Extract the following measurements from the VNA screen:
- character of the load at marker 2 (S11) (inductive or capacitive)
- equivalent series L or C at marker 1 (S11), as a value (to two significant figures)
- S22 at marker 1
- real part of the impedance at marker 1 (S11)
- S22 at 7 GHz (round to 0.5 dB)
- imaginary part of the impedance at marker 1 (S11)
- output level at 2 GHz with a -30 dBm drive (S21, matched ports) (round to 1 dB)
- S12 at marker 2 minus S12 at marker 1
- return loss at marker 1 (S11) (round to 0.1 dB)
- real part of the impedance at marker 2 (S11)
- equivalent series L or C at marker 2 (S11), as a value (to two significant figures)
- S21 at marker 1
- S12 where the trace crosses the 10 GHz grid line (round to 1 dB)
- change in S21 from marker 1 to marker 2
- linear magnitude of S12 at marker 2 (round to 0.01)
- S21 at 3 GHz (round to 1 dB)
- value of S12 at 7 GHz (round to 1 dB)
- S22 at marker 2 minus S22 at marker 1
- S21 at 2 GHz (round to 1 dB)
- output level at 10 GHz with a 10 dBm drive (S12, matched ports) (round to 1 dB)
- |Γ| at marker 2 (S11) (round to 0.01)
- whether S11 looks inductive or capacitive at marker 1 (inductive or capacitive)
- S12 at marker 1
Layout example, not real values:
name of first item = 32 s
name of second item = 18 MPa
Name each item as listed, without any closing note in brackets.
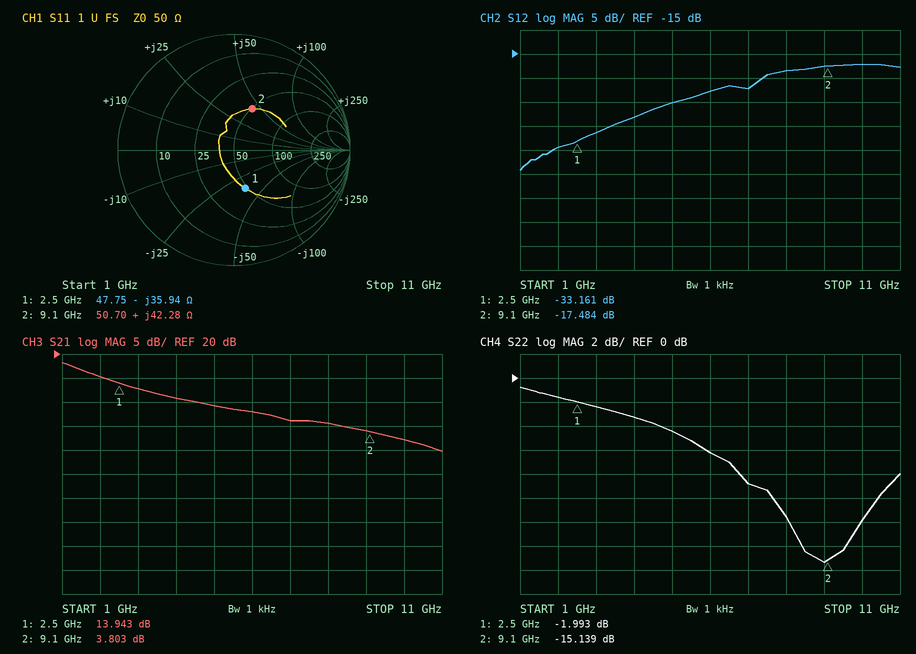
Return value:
character of the load at marker 2 (S11) = inductive
equivalent series L or C at marker 1 (S11), as a value = 1.8 pF
S22 at marker 1 = -1.993 dB
real part of the impedance at marker 1 = 47.75 Ω
S22 at 7 GHz = -9.0 dB
imaginary part of the impedance at marker 1 = -35.94 Ω
output level at 2 GHz with a -30 dBm drive (S21, matched ports) = -15 dBm
S12 at marker 2 minus S12 at marker 1 = 15.677 dB
return loss at marker 1 (S11) = 9.2 dB
real part of the impedance at marker 2 = 50.70 Ω
equivalent series L or C at marker 2 (S11), as a value = 740 pH
S21 at marker 1 = 13.943 dB
S12 where the trace crosses the 10 GHz grid line = -17 dB
change in S21 from marker 1 to marker 2 = -10.140 dB
linear magnitude of S12 at marker 2 = 0.13
S21 at 3 GHz = 13 dB
value of S12 at 7 GHz = -22 dB
S22 at marker 2 minus S22 at marker 1 = -13.146 dB
S21 at 2 GHz = 15 dB
output level at 10 GHz with a 10 dBm drive (S12, matched ports) = -7 dBm
|Γ| at marker 2 (S11) = 0.39
whether S11 looks inductive or capacitive at marker 1 = capacitive
S12 at marker 1 = -33.161 dB
